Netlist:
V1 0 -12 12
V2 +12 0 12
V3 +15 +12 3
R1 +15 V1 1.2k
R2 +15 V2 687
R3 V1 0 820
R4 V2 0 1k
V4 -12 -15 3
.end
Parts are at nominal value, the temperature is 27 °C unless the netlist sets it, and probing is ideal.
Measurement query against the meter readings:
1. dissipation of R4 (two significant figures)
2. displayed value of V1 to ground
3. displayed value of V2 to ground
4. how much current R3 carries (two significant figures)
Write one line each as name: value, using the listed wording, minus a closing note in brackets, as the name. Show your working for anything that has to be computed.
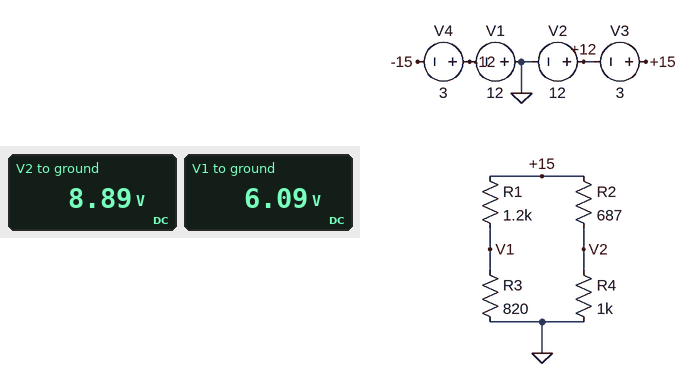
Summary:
dissipation of R4: (8.89 V)^2 / 1 kΩ = 79 mW
displayed value of V1 to ground: 6.09 V
displayed value of V2 to ground: 8.89 V
how much current R3 carries: (6.09 V) / 820 Ω = 7.4 mA
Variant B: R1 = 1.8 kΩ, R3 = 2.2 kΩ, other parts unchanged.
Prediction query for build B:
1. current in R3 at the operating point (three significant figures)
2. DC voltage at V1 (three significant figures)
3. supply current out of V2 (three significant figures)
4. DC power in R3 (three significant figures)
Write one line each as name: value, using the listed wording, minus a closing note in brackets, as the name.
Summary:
current in R3 at the operating point: 3.75 mA
DC voltage at V1: 8.25 V
supply current out of V2: 12.6 mA
DC power in R3: 30.9 mW
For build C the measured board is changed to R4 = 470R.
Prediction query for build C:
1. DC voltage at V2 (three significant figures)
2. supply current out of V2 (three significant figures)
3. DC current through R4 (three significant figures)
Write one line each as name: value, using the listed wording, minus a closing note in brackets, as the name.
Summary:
DC voltage at V2: 6.09 V
supply current out of V2: 20.4 mA
DC current through R4: 13.0 mA
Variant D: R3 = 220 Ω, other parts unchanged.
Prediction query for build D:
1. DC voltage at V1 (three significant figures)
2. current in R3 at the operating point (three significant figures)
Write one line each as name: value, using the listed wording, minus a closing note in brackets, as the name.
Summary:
DC voltage at V1: 2.32 V
current in R3 at the operating point: 10.6 mA
